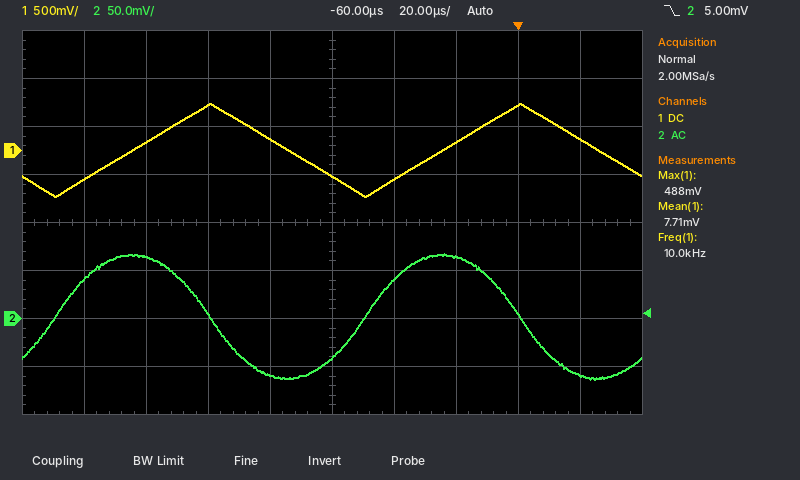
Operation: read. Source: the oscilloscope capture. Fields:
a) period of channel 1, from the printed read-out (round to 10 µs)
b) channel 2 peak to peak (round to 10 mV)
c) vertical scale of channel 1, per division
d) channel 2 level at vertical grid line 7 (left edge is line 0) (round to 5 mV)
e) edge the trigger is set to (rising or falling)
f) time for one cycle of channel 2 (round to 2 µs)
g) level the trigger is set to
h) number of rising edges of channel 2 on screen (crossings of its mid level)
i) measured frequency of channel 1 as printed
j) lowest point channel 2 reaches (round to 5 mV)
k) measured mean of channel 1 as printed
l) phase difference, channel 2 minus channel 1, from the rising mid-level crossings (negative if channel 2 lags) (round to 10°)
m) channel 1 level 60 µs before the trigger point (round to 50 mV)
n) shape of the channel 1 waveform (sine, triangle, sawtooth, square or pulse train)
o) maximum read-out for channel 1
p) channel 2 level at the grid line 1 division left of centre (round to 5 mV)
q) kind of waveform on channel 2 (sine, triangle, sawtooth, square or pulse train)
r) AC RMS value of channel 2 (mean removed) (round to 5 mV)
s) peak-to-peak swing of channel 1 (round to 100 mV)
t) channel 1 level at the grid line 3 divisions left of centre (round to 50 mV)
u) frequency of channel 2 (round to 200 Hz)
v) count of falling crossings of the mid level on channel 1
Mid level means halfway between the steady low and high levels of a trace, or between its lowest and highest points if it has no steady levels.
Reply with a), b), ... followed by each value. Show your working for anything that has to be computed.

a) 1 / 10.0 kHz ≈ 100 µs
b) 130 mV
c) 500 mV
d) 65 mV
e) falling
f) 100 µs
g) 5.00 mV
h) 2
i) 10.0 kHz
j) -65 mV
k) 7.71 mV
l) +90°
m) -250 mV
n) triangle
o) 488 mV
p) -60 mV
q) sine
r) 130 mV / (2√2) ≈ 46.0 mV, so 45 mV to the nearest 5 mV
s) 1.00 V
t) 100 mV
u) 1 / 100 µs ≈ 10.0 kHz
v) 2
